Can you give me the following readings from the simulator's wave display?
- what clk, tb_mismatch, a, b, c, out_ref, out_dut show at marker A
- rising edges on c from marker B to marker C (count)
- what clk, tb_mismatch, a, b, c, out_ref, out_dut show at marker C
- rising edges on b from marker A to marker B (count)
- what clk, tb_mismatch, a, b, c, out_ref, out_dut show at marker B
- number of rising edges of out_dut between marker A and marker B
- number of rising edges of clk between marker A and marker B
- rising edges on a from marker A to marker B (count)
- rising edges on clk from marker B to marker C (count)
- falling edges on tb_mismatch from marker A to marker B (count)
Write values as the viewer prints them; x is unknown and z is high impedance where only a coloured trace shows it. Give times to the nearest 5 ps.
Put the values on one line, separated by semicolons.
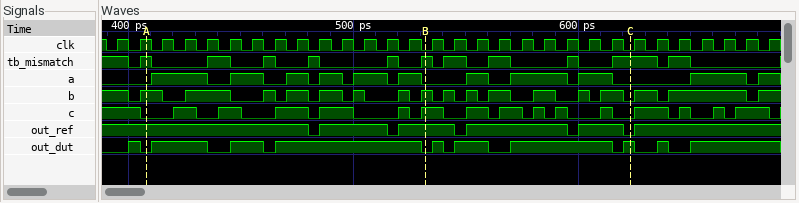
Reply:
clk=1, tb_mismatch=1, a=0, b=1, c=0, out_ref=1, out_dut=0; 5; clk=0, tb_mismatch=1, a=0, b=0, c=0, out_ref=0, out_dut=1; 7; clk=0, tb_mismatch=1, a=0, b=1, c=1, out_ref=1, out_dut=0; 3; 12; 6; 9; 5
